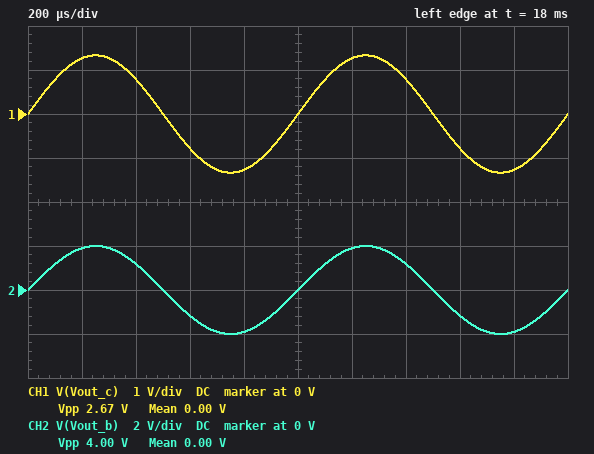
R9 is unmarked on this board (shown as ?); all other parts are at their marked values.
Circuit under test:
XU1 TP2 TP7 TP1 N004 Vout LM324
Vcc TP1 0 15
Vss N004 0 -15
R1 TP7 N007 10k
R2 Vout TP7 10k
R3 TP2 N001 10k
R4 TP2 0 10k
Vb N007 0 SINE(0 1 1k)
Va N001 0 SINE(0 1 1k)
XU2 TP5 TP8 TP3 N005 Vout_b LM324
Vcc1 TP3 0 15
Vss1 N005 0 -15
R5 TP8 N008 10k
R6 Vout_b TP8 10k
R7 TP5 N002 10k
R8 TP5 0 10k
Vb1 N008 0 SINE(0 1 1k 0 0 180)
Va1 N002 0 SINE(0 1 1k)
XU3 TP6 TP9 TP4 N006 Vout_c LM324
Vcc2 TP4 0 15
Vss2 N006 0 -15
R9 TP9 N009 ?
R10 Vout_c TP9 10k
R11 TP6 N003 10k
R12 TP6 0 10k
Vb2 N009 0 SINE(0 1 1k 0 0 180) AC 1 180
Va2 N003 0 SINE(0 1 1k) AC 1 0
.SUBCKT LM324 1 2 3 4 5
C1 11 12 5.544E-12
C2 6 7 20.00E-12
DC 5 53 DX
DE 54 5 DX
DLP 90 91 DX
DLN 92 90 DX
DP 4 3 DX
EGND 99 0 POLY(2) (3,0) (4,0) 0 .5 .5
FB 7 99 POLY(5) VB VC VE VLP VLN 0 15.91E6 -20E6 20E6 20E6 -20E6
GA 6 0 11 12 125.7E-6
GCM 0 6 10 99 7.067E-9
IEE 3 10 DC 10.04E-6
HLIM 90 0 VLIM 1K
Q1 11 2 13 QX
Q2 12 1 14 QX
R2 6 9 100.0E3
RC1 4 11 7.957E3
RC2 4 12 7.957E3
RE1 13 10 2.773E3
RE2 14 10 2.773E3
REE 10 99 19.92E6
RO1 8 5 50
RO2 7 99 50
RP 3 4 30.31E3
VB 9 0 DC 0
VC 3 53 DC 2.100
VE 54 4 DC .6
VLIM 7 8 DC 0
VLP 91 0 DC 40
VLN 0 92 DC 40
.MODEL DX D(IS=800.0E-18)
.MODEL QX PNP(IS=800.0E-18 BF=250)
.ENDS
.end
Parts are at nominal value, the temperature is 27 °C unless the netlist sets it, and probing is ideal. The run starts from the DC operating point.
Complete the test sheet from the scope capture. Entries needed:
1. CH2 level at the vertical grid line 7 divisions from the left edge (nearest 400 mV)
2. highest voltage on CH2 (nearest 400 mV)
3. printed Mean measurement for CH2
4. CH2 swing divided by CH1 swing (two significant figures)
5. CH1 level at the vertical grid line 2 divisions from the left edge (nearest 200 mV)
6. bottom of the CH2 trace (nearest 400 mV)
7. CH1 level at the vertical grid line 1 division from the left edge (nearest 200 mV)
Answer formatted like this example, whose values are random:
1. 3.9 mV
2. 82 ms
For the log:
1. 1.2 V
2. 2.0 V
3. 0.00 V
4. 1.5
5. 800 mV
6. -2.0 V
7. 1.2 V
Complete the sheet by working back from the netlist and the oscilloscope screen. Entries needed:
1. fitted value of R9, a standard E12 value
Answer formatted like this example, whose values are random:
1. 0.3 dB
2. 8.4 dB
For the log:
1. 18 kΩ
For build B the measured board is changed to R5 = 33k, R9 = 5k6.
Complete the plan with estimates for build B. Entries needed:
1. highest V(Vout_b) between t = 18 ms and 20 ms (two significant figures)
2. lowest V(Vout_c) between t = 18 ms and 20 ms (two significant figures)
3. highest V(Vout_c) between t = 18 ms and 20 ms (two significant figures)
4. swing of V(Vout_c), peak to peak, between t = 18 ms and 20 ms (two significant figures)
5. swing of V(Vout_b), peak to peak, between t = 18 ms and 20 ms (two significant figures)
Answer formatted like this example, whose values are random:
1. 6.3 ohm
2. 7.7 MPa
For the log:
1. 950 mV
2. -3.2 V
3. 3.2 V
4. 6.4 V
5. 1.9 V
